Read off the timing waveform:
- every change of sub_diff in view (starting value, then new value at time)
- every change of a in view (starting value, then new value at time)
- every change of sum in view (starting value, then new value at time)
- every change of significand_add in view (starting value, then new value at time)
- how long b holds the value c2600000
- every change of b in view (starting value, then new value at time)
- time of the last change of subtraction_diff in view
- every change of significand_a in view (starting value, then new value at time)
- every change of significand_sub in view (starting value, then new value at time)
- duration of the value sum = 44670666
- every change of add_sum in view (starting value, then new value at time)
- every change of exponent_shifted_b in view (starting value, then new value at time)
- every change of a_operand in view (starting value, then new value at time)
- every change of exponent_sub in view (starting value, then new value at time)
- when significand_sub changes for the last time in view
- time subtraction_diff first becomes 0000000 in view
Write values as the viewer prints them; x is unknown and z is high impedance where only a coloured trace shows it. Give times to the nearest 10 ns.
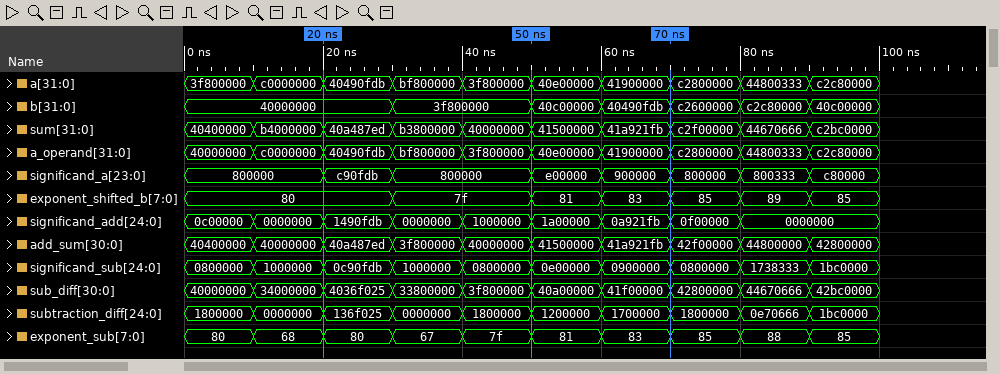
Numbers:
40000000, 34000000 at 10 ns, 4036f025 at 20 ns, 33800000 at 30 ns, 3f800000 at 40 ns, 40a00000 at 50 ns, 41f00000 at 60 ns, 42800000 at 70 ns, 44670666 at 80 ns, 42bc0000 at 90 ns
3f800000, c0000000 at 10 ns, 40490fdb at 20 ns, bf800000 at 30 ns, 3f800000 at 40 ns, 40e00000 at 50 ns, 41900000 at 60 ns, c2800000 at 70 ns, 44800333 at 80 ns, c2c80000 at 90 ns
40400000, b4000000 at 10 ns, 40a487ed at 20 ns, b3800000 at 30 ns, 40000000 at 40 ns, 41500000 at 50 ns, 41a921fb at 60 ns, c2f00000 at 70 ns, 44670666 at 80 ns, c2bc0000 at 90 ns
0c00000, 0000000 at 10 ns, 1490fdb at 20 ns, 0000000 at 30 ns, 1000000 at 40 ns, 1a00000 at 50 ns, 0a921fb at 60 ns, 0f00000 at 70 ns, 0000000 at 80 ns
10 ns
40000000, 3f800000 at 30 ns, 40c00000 at 50 ns, 40490fdb at 60 ns, c2600000 at 70 ns, c2c80000 at 80 ns, 40c00000 at 90 ns
90 ns
800000, c90fdb at 20 ns, 800000 at 30 ns, e00000 at 50 ns, 900000 at 60 ns, 800000 at 70 ns, 800333 at 80 ns, c80000 at 90 ns
0800000, 1000000 at 10 ns, 0c90fdb at 20 ns, 1000000 at 30 ns, 0800000 at 40 ns, 0e00000 at 50 ns, 0900000 at 60 ns, 0800000 at 70 ns, 1738333 at 80 ns, 1bc0000 at 90 ns
10 ns
40400000, 40000000 at 10 ns, 40a487ed at 20 ns, 3f800000 at 30 ns, 40000000 at 40 ns, 41500000 at 50 ns, 41a921fb at 60 ns, 42f00000 at 70 ns, 44800000 at 80 ns, 42800000 at 90 ns
80, 7f at 30 ns, 81 at 50 ns, 83 at 60 ns, 85 at 70 ns, 89 at 80 ns, 85 at 90 ns
40000000, c0000000 at 10 ns, 40490fdb at 20 ns, bf800000 at 30 ns, 3f800000 at 40 ns, 40e00000 at 50 ns, 41900000 at 60 ns, c2800000 at 70 ns, 44800333 at 80 ns, c2c80000 at 90 ns
80, 68 at 10 ns, 80 at 20 ns, 67 at 30 ns, 7f at 40 ns, 81 at 50 ns, 83 at 60 ns, 85 at 70 ns, 88 at 80 ns, 85 at 90 ns
90 ns
10 ns
